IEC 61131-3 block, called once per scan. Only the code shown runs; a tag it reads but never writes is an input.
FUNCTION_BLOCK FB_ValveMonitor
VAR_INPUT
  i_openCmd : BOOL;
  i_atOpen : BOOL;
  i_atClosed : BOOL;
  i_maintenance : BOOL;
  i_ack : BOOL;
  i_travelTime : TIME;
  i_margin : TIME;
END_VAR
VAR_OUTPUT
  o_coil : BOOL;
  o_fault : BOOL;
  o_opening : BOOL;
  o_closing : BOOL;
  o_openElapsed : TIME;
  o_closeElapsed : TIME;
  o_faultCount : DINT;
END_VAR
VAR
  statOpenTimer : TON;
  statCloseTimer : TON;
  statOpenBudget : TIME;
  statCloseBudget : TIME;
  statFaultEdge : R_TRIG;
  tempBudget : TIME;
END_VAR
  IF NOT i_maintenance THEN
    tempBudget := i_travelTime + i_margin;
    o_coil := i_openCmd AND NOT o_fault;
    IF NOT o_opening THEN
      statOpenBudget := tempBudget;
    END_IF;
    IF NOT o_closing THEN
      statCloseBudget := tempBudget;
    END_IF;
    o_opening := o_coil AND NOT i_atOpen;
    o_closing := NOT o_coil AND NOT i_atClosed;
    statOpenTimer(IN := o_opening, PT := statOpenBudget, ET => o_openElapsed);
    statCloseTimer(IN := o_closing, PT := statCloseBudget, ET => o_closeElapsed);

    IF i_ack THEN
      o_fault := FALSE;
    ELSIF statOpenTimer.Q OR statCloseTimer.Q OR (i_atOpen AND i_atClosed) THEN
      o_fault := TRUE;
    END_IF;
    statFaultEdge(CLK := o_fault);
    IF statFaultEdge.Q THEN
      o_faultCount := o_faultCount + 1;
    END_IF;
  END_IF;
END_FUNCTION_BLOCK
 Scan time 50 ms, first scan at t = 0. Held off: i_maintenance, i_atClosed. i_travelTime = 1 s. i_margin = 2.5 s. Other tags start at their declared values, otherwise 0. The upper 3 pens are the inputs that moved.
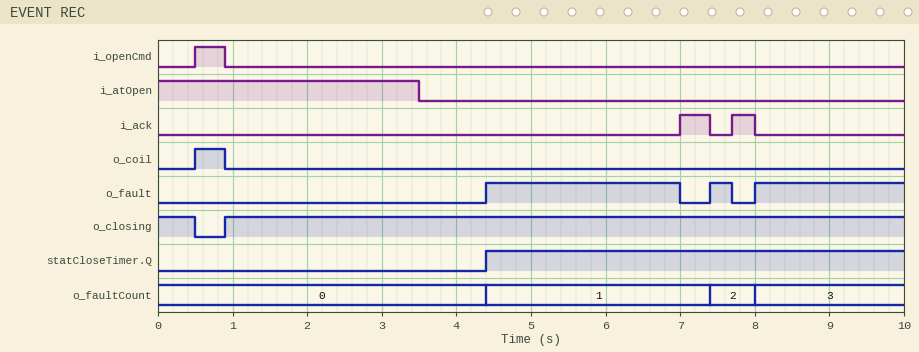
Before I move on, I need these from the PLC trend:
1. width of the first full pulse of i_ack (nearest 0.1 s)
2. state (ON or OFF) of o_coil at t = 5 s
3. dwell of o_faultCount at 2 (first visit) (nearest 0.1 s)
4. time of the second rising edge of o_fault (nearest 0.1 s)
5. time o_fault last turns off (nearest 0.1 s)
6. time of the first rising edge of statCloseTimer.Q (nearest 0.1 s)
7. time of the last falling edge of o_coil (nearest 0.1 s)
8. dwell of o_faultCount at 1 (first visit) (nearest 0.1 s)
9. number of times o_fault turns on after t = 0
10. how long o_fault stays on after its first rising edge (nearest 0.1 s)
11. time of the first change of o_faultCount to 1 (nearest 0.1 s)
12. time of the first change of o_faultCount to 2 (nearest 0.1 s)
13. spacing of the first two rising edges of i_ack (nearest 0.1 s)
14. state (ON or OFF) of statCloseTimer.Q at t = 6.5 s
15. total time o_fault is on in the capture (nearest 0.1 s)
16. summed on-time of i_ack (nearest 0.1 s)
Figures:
0.4 s
OFF
0.6 s
7.4 s
7.7 s
4.4 s
0.9 s
3.0 s
3
2.6 s
4.4 s
7.4 s
0.7 s
ON
4.9 s
0.7 s
